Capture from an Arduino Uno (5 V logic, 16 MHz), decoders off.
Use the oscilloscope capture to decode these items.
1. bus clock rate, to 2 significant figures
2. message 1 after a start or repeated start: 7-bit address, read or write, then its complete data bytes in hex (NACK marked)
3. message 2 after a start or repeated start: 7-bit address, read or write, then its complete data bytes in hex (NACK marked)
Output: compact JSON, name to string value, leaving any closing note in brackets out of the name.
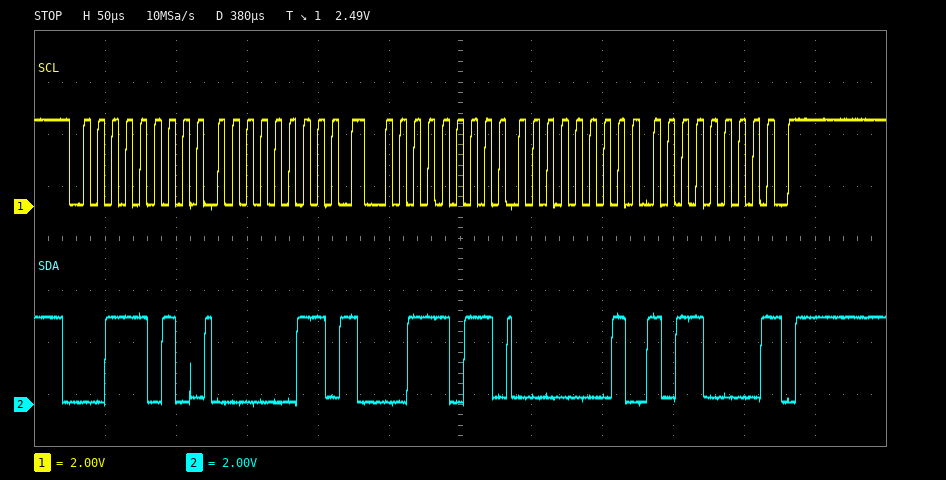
{"bus clock rate, to 2 significant figures": "100 kHz", "message 1 after a start or repeated start: 7-bit address, read or write, then its complete data bytes in hex": "0x1D write: 03", "message 2 after a start or repeated start: 7-bit address, read or write, then its complete data bytes in hex": "0x1D read: 01 B0 NACK"}
